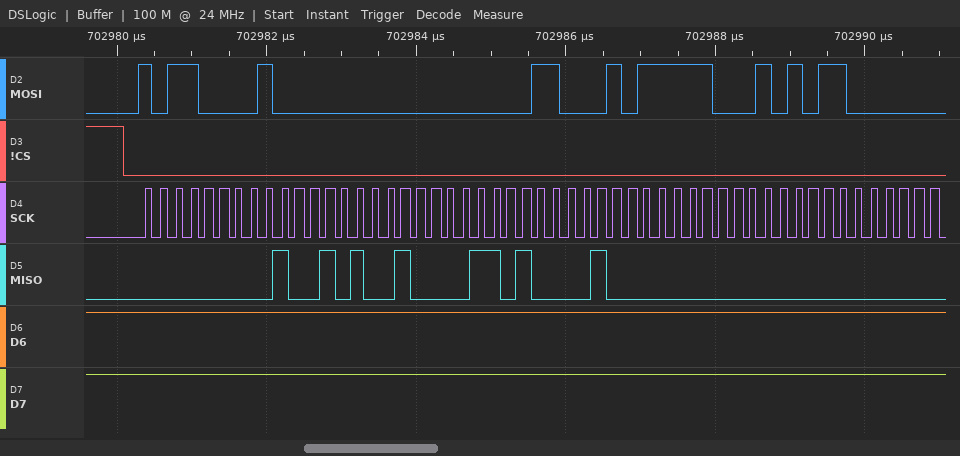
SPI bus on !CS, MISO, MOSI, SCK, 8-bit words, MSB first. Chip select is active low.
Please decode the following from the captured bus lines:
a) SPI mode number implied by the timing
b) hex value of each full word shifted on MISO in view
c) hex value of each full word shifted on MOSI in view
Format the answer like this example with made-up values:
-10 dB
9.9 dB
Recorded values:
0
00, 4A, 43, 42, 00, 00
B0, 80, 00, 31, 7C, 56
